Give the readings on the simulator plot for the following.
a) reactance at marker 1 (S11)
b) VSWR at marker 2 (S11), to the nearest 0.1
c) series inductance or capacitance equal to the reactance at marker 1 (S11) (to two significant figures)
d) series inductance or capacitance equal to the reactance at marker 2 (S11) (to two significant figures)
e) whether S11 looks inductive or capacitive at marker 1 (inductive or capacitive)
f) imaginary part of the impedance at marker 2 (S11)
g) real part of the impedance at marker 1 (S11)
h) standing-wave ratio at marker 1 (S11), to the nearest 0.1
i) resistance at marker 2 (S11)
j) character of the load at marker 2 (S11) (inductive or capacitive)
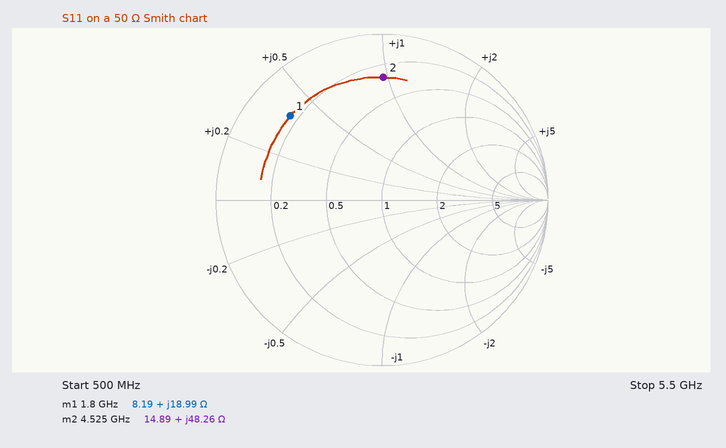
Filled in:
+18.99 Ω
6.6
1.7 nH
1.7 nH
inductive
+48.26 Ω
8.19 Ω
7.0
14.89 Ω
inductive
